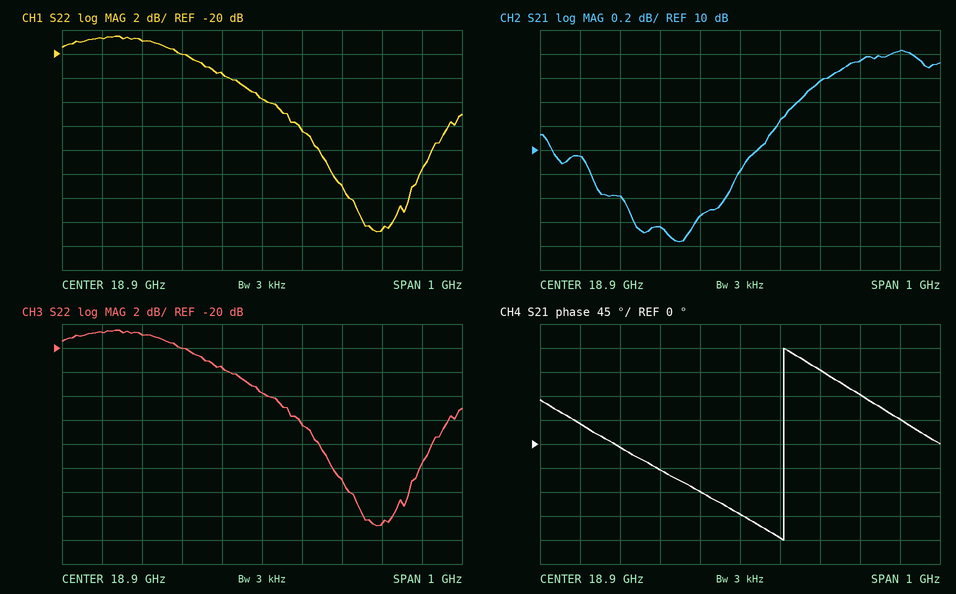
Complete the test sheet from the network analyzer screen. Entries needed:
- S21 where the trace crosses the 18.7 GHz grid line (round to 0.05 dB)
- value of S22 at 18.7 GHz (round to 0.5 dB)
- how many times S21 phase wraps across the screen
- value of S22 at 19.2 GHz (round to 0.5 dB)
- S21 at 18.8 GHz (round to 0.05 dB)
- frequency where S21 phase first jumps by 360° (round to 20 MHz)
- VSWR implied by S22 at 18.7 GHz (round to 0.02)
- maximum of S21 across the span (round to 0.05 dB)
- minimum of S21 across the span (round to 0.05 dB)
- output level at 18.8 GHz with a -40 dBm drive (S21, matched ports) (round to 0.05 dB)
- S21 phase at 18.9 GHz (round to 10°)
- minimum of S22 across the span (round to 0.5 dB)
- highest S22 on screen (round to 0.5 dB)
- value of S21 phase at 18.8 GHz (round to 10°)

9.35 dB
-20.0 dB
1
-34.5 dB
9.45 dB
19.00 GHz
1.22
10.85 dB
9.25 dB
-30.55 dBm
-130°
-35.0 dB
-18.5 dB
-90°
